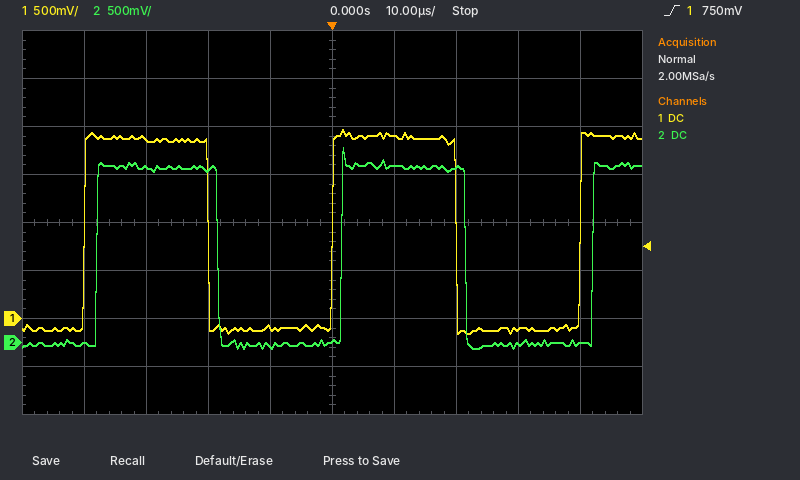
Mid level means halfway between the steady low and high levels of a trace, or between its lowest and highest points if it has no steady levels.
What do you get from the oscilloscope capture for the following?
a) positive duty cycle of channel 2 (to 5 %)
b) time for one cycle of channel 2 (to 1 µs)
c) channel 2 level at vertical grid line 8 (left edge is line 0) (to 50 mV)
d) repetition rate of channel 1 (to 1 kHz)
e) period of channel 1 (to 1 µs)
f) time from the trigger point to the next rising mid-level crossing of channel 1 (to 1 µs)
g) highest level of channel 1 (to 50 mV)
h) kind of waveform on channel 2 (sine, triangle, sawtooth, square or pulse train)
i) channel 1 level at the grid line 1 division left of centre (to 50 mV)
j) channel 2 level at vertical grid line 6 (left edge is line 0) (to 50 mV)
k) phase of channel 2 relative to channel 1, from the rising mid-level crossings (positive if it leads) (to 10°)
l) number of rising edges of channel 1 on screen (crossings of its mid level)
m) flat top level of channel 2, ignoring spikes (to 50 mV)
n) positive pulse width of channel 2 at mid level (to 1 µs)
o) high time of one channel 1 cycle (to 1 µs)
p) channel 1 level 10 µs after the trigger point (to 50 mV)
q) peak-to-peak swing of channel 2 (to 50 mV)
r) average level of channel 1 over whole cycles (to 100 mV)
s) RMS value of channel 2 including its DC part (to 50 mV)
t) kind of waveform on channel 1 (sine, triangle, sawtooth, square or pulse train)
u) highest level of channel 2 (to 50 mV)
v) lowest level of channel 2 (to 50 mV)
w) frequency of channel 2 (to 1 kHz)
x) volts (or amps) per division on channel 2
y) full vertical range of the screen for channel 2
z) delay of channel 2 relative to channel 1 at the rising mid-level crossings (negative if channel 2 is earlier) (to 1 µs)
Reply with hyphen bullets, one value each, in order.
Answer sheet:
- 50 %
- 40 µs
- 0 mV
- 25 kHz
- 40 µs
- 40 µs
- 1.95 V
- square
- -100 mV
- 1.85 V
- -20°
- 3
- 1.85 V
- 20 µs
- 20 µs
- 1.90 V
- 2.10 V
- 900 mV
- 1.30 V
- square
- 2.05 V
- -50 mV
- 25 kHz
- 500 mV
- 4 V
- +2 µs
